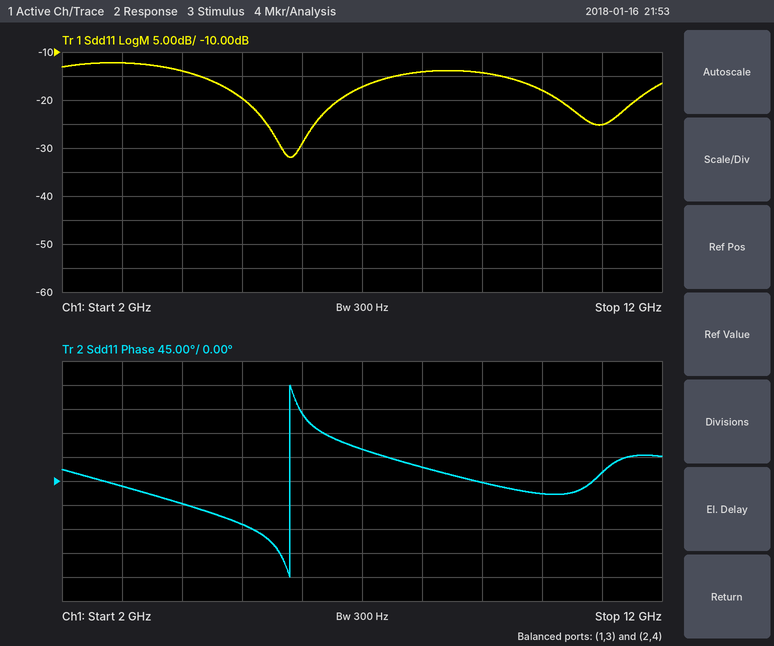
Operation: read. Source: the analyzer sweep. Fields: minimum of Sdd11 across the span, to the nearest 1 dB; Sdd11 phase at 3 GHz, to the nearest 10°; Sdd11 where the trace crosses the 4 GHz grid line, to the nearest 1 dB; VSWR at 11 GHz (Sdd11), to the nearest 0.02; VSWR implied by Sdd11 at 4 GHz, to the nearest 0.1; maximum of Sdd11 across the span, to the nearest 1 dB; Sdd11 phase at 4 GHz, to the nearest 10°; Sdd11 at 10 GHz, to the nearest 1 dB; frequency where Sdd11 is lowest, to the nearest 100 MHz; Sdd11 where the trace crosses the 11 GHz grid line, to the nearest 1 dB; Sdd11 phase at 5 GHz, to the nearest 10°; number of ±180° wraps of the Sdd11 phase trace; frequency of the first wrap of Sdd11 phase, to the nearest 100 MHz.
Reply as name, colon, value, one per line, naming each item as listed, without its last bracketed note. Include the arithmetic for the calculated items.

minimum of Sdd11 across the span, to the nearest 1 dB: -32 dB
Sdd11 phase at 3 GHz, to the nearest 10°: -10°
Sdd11 where the trace crosses the 4 GHz grid line, to the nearest 1 dB: -14 dB
VSWR at 11 GHz (Sdd11), to the nearest 0.02: |Γ| = 10^(-25/20) = 0.0562; VSWR = (1 + 0.0562)/(1 − 0.0562) ≈ 1.12
VSWR implied by Sdd11 at 4 GHz, to the nearest 0.1: |Γ| = 10^(-14/20) = 0.1995; VSWR = (1 + 0.1995)/(1 − 0.1995) ≈ 1.5
maximum of Sdd11 across the span, to the nearest 1 dB: -12 dB
Sdd11 phase at 4 GHz, to the nearest 10°: -40°
Sdd11 at 10 GHz, to the nearest 1 dB: -18 dB
frequency where Sdd11 is lowest, to the nearest 100 MHz: 5.8 GHz
Sdd11 where the trace crosses the 11 GHz grid line, to the nearest 1 dB: -25 dB
Sdd11 phase at 5 GHz, to the nearest 10°: -80°
number of ±180° wraps of the Sdd11 phase trace: 1
frequency of the first wrap of Sdd11 phase, to the nearest 100 MHz: 5.8 GHz
